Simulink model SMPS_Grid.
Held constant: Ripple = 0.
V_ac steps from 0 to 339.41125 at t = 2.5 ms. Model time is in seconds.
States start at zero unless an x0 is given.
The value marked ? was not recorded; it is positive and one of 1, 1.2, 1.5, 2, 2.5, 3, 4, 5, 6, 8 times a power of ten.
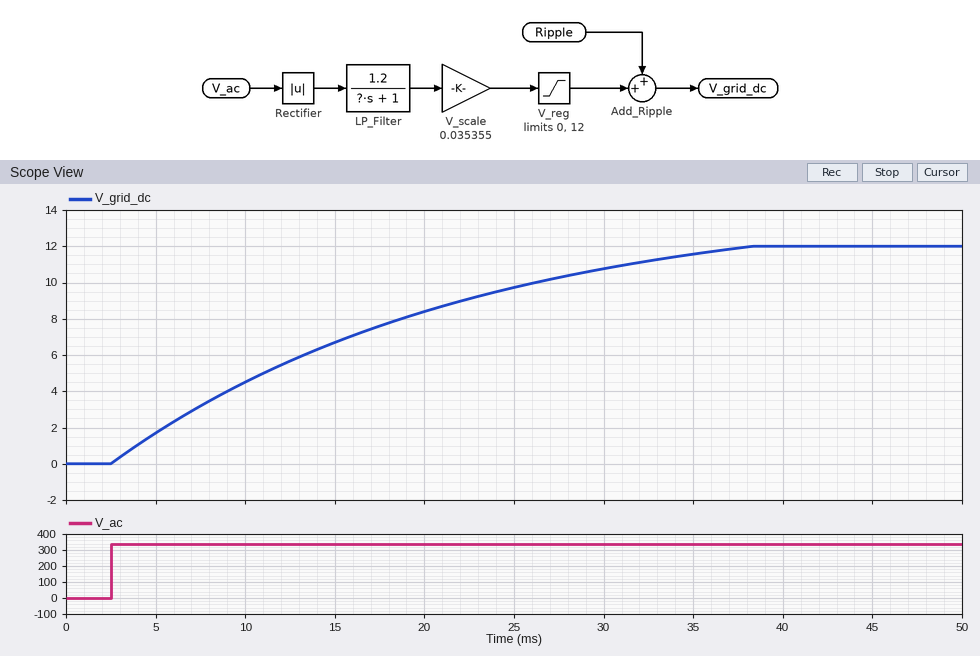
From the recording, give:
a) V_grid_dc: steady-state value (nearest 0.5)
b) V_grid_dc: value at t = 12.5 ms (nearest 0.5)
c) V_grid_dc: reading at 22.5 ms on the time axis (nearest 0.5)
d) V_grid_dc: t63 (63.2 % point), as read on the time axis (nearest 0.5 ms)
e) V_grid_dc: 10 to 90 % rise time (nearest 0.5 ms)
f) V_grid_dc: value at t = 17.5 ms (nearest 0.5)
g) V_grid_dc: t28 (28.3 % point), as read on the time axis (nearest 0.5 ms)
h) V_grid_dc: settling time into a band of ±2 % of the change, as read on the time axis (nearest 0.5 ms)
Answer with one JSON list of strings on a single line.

["12.0", "5.5", "9.0", "17.5 ms", "26.0 ms", "7.5", "8.0 ms", "36.5 ms"]
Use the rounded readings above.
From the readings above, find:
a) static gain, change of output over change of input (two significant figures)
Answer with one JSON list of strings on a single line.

["0.035"]
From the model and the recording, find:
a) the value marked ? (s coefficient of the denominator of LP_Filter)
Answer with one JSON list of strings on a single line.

["0.02"]
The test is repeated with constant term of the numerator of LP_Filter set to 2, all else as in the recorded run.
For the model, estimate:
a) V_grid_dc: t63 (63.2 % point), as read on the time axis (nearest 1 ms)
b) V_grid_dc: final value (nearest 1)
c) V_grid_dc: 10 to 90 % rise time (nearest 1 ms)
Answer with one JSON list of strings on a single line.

["10 ms", "12", "11 ms"]
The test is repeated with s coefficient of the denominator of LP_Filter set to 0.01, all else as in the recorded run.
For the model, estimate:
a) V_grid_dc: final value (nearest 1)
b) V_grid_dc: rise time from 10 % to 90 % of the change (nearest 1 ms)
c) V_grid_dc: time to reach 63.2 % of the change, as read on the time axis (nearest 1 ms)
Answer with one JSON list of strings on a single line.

["12", "13 ms", "10 ms"]
